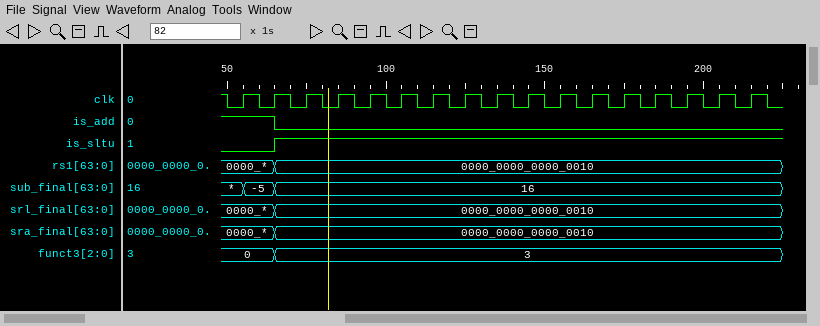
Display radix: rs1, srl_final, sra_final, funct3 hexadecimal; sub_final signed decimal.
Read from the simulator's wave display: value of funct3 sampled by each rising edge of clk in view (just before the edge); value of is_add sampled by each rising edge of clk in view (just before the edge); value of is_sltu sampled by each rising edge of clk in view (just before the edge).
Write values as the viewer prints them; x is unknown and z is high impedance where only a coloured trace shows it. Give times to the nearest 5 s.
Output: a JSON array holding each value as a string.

["0, 0, 3, 3, 3, 3, 3, 3, 3, 3, 3, 3, 3, 3, 3, 3, 3", "1 1 0 0 0 0 0 0 0 0 0 0 0 0 0 0 0", "0 0 1 1 1 1 1 1 1 1 1 1 1 1 1 1 1"]
